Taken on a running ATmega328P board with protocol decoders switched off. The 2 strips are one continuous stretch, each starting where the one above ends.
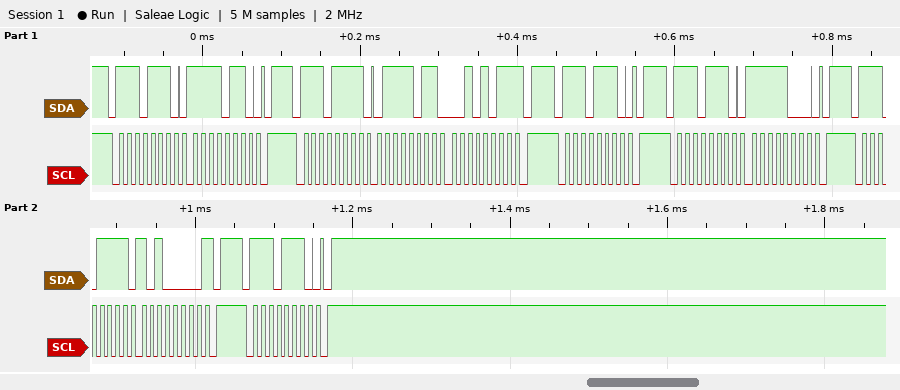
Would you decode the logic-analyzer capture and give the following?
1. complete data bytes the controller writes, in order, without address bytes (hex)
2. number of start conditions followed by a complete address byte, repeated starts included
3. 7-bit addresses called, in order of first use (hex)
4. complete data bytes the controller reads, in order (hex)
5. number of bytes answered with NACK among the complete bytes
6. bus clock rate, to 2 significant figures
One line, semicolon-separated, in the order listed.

F6 F8; 6; 0x77; 7B 2B A0; 2; 100 kHz
